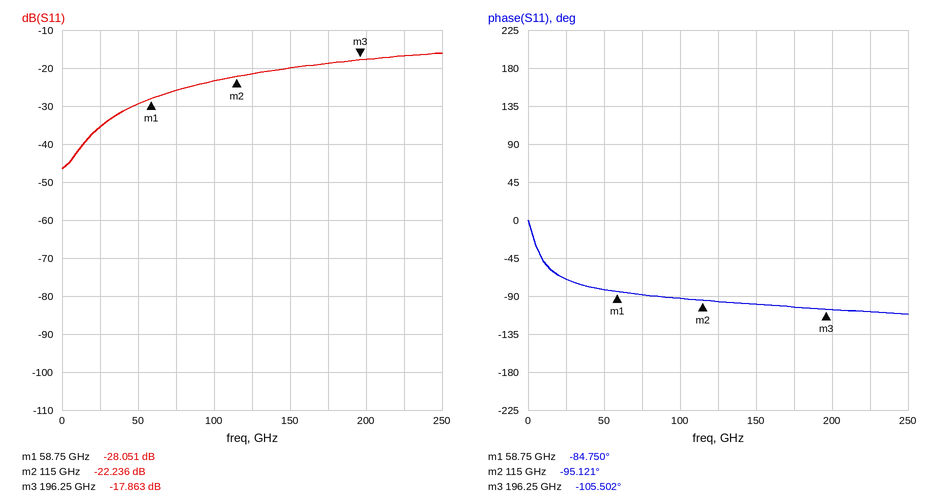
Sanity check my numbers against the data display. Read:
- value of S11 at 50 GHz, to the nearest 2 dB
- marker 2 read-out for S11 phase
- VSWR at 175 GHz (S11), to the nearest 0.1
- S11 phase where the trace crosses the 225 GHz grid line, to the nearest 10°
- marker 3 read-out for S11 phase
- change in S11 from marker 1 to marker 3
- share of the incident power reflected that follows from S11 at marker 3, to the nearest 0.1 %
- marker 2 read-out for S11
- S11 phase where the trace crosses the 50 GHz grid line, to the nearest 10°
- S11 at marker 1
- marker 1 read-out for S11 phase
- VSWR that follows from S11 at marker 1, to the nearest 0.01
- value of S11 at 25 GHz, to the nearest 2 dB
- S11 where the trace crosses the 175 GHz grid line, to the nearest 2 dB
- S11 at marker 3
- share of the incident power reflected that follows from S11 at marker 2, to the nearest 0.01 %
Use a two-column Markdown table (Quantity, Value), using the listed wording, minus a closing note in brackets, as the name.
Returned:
| Quantity | Value |
|---|---|
| value of S11 at 50 GHz, to the nearest 2 dB | -30 dB |
| marker 2 read-out for S11 phase | -95.121° |
| VSWR at 175 GHz (S11), to the nearest 0.1 | 1.3 |
| S11 phase where the trace crosses the 225 GHz grid line, to the nearest 10° | -110° |
| marker 3 read-out for S11 phase | -105.502° |
| change in S11 from marker 1 to marker 3 | 10.188 dB |
| share of the incident power reflected that follows from S11 at marker 3, to the nearest 0.1 % | 1.6 % |
| marker 2 read-out for S11 | -22.236 dB |
| S11 phase where the trace crosses the 50 GHz grid line, to the nearest 10° | -80° |
| S11 at marker 1 | -28.051 dB |
| marker 1 read-out for S11 phase | -84.750° |
| VSWR that follows from S11 at marker 1, to the nearest 0.01 | 1.08 |
| value of S11 at 25 GHz, to the nearest 2 dB | -36 dB |
| S11 where the trace crosses the 175 GHz grid line, to the nearest 2 dB | -18 dB |
| S11 at marker 3 | -17.863 dB |
| share of the incident power reflected that follows from S11 at marker 2, to the nearest 0.01 % | 0.60 % |
